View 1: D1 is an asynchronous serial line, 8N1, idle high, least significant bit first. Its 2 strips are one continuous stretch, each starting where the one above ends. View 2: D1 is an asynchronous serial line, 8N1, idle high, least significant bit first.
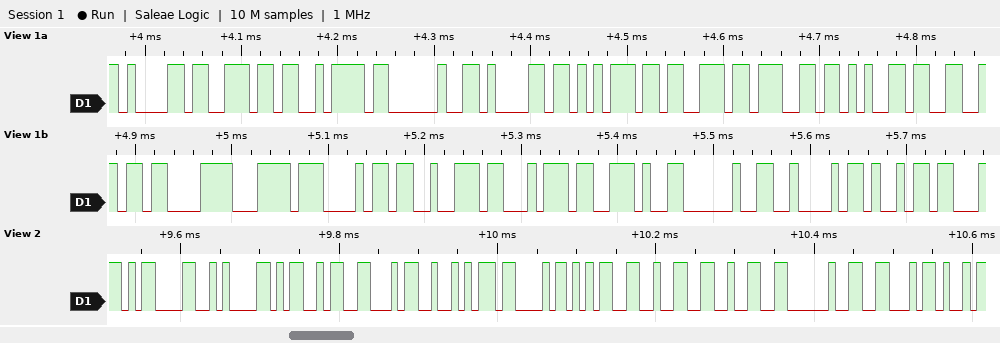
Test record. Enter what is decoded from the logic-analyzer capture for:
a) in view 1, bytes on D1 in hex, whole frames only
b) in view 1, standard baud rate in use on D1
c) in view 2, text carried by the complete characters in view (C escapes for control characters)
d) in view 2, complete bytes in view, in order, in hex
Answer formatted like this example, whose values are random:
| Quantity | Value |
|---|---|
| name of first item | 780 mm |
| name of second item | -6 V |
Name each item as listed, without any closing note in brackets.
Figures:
| Quantity | Value |
|---|---|
| in view 1, bytes on D1 in hex, whole frames only | 61 6E 7A 20 61 75 73 67 65 66 C3 BC 68 72 74 2E 20 42 69 |
| in view 1, standard baud rate in use on D1 | 115200 baud |
| in view 2, text carried by the complete characters in view | "\r\nMFRC522 F" |
| in view 2, complete bytes in view, in order, in hex | 0D 0A 4D 46 52 43 35 32 32 20 46 |
